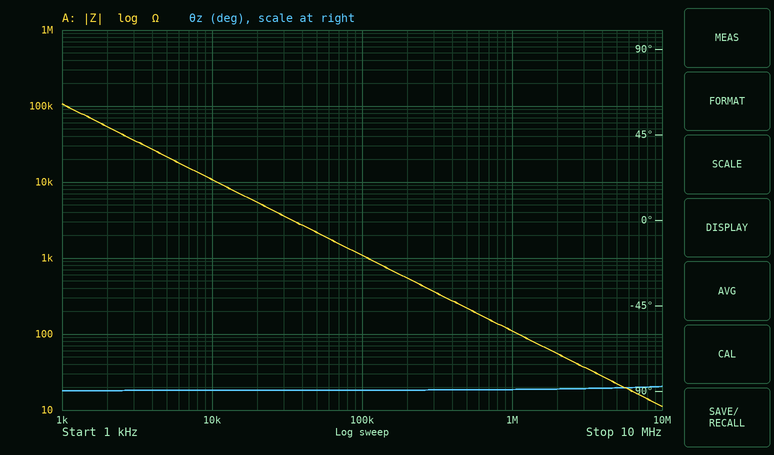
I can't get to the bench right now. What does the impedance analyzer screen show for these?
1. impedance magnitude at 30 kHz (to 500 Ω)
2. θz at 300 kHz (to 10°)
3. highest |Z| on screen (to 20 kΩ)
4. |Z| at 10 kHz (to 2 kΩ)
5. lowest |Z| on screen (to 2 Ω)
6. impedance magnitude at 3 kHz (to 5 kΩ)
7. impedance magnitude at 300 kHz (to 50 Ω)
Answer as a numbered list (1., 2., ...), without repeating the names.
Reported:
1. 3.5 kΩ
2. -90°
3. 100 kΩ
4. 10 kΩ
5. 12 Ω
6. 35 kΩ
7. 350 Ω
